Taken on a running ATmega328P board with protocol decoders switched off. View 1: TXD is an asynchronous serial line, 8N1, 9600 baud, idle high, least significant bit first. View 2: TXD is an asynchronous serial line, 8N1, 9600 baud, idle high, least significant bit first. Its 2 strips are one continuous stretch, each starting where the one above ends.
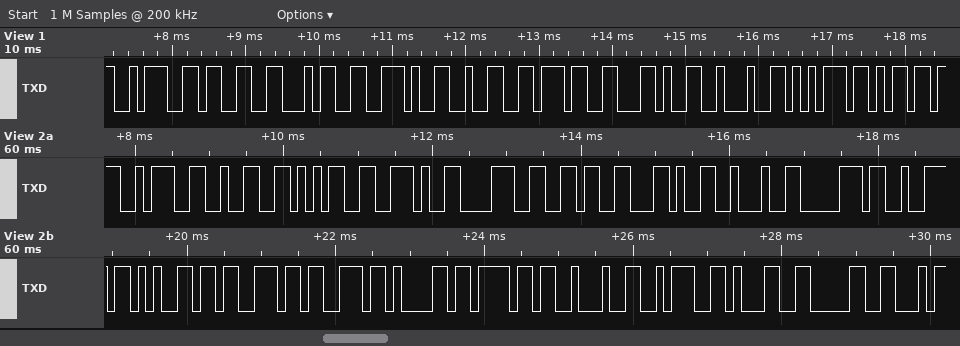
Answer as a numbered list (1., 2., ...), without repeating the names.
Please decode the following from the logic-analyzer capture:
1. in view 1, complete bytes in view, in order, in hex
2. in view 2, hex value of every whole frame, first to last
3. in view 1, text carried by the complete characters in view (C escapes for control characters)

1. 3A 33 34 2E 32 37 2C 22 75 6D
2. 3A 32 35 2E 38 36 2C 22 70 72 65 73 73 61 6F 22 3A 31 30
3. ":34.27,\"um"
